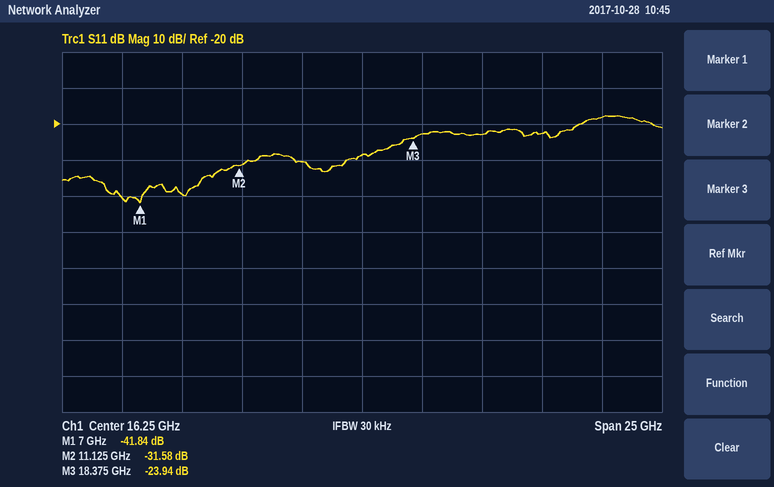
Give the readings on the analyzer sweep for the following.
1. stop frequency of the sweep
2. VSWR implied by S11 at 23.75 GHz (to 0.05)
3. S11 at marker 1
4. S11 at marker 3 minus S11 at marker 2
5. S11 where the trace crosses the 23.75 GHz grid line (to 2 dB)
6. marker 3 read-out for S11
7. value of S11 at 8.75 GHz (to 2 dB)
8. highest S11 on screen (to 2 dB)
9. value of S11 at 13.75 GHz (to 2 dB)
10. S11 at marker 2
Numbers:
28.75 GHz
1.15
-41.84 dB
7.64 dB
-22 dB
-23.94 dB
-40 dB
-18 dB
-30 dB
-31.58 dB
